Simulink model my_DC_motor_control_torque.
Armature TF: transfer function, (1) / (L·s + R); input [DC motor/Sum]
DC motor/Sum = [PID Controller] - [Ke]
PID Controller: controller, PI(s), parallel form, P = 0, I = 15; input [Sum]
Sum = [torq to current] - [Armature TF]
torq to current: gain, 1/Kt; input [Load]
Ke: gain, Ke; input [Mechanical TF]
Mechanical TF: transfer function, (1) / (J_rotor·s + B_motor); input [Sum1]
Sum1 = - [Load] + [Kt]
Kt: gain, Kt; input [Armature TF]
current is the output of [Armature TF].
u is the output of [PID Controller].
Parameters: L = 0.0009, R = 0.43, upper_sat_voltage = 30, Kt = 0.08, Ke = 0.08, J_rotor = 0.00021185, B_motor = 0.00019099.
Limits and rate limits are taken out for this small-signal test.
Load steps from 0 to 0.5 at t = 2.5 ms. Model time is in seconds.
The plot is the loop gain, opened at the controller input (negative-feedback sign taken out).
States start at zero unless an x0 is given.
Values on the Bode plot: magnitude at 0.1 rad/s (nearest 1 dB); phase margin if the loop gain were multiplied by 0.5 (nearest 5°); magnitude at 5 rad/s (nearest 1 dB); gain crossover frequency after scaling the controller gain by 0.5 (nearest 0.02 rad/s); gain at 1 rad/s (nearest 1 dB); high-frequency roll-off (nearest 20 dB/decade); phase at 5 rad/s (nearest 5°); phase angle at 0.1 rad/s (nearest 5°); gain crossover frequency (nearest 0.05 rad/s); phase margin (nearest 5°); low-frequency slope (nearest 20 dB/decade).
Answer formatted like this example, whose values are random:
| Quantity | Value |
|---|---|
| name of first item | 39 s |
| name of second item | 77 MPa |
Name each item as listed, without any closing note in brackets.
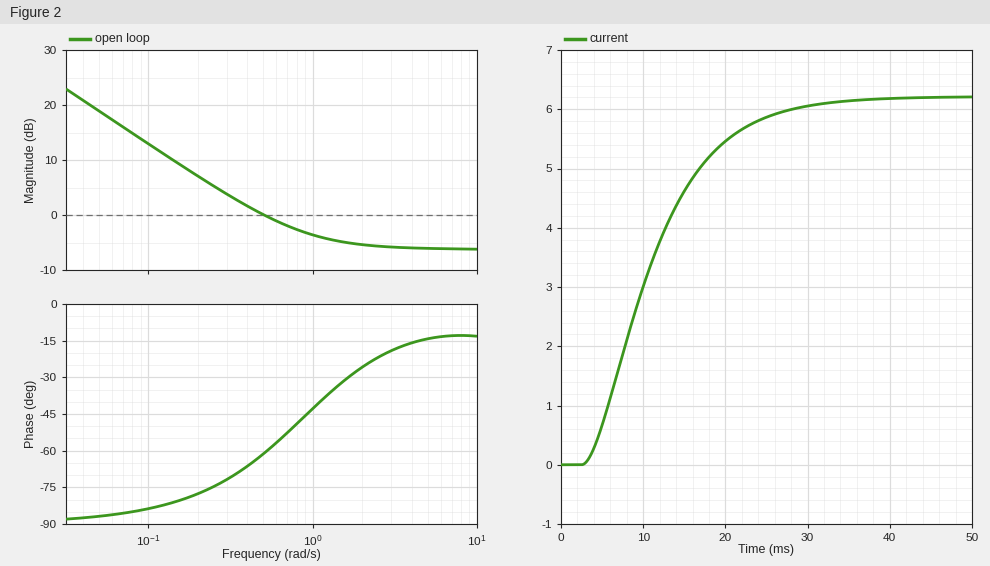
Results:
| Quantity | Value |
|---|---|
| magnitude at 0.1 rad/s | 13 dB |
| phase margin if the loop gain were multiplied by 0.5 | 105° |
| magnitude at 5 rad/s | -6 dB |
| gain crossover frequency after scaling the controller gain by 0.5 | 0.22 rad/s |
| gain at 1 rad/s | -4 dB |
| high-frequency roll-off | 0 dB/decade |
| phase at 5 rad/s | -15° |
| phase angle at 0.1 rad/s | -85° |
| gain crossover frequency | 0.50 rad/s |
| phase margin | 120° |
| low-frequency slope | -20 dB/decade |
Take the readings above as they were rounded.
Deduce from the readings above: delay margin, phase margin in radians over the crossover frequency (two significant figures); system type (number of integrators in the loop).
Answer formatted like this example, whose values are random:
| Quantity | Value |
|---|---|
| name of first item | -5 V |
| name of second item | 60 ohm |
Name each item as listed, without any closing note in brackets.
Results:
| Quantity | Value |
|---|---|
| delay margin, phase margin in radians over the crossover frequency | 4.2 s |
| system type | 1 |
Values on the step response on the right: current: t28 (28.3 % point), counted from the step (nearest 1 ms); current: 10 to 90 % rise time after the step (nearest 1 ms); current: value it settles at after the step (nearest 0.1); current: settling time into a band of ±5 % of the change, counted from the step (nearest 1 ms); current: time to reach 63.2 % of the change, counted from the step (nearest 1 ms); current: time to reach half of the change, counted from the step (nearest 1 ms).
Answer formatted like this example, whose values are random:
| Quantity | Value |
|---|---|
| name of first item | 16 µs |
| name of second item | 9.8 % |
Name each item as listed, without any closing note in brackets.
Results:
| Quantity | Value |
|---|---|
| current: t28 (28.3 % point), counted from the step | 5 ms |
| current: 10 to 90 % rise time after the step | 16 ms |
| current: value it settles at after the step | 6.2 |
| current: settling time into a band of ±5 % of the change, counted from the step | 23 ms |
| current: time to reach 63.2 % of the change, counted from the step | 10 ms |
| current: time to reach half of the change, counted from the step | 8 ms |
